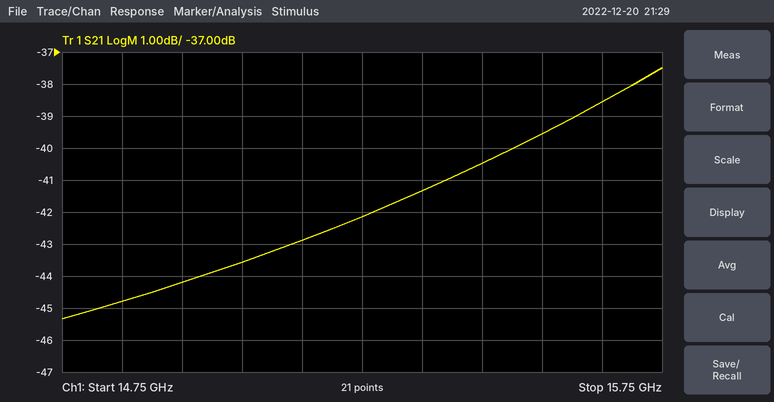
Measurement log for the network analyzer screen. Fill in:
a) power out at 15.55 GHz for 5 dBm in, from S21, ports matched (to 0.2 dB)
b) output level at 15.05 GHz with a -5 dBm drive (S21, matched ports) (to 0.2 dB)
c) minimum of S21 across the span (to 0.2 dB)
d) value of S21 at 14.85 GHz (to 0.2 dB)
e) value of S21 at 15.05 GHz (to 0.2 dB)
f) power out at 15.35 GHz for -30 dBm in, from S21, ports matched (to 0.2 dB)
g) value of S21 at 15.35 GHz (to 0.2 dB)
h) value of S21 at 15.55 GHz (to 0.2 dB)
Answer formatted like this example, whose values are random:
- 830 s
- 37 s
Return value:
- -34.6 dBm
- -48.6 dBm
- -45.4 dB
- -44.8 dB
- -43.6 dB
- -71.4 dBm
- -41.4 dB
- -39.6 dB
